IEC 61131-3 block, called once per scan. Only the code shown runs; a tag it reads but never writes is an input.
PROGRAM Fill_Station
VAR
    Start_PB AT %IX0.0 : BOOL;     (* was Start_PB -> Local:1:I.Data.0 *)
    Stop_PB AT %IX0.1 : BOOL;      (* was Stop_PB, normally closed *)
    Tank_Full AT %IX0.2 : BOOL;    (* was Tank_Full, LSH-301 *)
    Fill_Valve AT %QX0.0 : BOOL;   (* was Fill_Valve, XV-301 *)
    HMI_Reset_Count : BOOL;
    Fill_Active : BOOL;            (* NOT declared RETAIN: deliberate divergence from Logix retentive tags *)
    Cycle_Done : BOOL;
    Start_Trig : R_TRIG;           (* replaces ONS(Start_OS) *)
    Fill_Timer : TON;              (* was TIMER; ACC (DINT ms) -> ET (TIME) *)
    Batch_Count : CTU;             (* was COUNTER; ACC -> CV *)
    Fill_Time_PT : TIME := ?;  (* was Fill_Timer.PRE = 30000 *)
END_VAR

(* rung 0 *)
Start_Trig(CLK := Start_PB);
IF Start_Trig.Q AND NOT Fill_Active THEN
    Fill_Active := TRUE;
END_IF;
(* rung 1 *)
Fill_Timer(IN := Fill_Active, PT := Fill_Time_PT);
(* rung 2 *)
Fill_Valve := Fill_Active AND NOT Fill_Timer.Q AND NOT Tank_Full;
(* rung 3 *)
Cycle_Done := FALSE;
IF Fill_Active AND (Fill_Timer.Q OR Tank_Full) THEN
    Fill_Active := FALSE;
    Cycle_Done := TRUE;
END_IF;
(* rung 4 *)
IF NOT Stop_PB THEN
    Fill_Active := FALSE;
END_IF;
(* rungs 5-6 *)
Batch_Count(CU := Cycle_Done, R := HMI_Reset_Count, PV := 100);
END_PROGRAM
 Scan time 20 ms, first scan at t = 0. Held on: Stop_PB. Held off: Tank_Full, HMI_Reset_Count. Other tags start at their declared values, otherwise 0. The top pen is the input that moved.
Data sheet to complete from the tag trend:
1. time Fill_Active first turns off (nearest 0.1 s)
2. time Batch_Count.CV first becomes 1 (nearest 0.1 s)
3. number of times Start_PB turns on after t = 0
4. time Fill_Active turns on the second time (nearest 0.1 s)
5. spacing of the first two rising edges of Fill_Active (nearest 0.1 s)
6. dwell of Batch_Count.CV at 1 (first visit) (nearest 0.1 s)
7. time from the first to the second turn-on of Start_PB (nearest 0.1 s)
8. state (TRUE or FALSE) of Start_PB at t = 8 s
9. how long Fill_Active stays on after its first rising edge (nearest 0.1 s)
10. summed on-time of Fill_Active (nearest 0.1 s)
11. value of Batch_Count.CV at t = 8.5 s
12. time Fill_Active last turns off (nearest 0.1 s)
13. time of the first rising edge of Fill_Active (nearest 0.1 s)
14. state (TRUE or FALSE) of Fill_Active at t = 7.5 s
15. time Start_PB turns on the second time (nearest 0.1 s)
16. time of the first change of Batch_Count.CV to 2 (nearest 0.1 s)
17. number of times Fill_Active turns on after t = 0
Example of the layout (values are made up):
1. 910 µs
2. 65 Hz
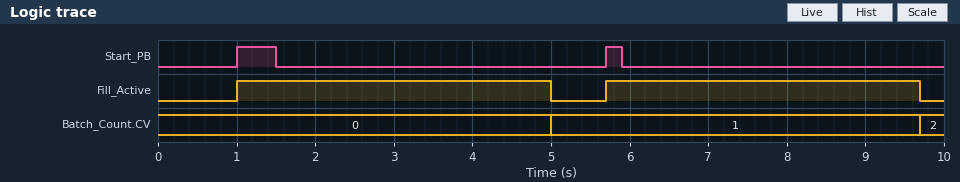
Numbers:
1. 5.0 s
2. 5.0 s
3. 2
4. 5.7 s
5. 4.7 s
6. 4.7 s
7. 4.7 s
8. FALSE
9. 4.0 s
10. 8.0 s
11. 1
12. 9.7 s
13. 1.0 s
14. TRUE
15. 5.7 s
16. 9.7 s
17. 2
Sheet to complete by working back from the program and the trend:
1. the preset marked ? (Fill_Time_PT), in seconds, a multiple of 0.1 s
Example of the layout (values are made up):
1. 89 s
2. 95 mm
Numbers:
1. 4.0 s
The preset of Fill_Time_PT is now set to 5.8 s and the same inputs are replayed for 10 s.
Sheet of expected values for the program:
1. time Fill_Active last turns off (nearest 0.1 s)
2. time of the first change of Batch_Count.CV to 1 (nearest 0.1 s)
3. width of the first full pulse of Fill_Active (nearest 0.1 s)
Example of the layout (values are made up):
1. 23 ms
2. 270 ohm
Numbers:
1. 6.8 s
2. 6.8 s
3. 5.8 s
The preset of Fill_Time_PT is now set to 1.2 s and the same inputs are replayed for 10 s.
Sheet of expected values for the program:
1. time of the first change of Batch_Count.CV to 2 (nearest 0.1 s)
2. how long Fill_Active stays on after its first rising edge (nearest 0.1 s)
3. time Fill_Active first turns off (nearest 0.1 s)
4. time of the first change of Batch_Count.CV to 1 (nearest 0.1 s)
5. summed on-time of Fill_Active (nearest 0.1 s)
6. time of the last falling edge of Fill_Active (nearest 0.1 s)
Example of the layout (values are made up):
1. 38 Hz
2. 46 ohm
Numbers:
1. 6.9 s
2. 1.2 s
3. 2.2 s
4. 2.2 s
5. 2.4 s
6. 6.9 s
